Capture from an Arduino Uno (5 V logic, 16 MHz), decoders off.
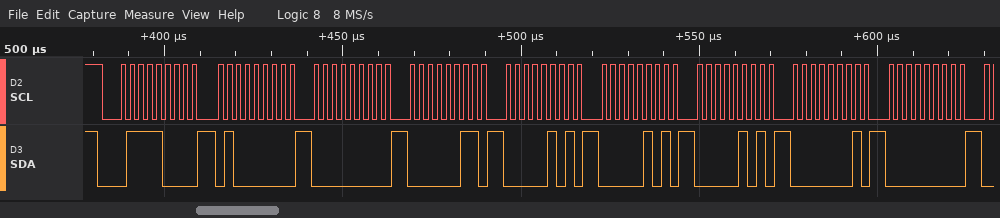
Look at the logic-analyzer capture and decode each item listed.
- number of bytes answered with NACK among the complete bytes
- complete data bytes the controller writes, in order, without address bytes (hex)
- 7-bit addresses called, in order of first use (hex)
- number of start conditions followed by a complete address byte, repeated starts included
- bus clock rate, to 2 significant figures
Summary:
0
40 00 03 05 05 05 01 00
0x3C
1
400 kHz
